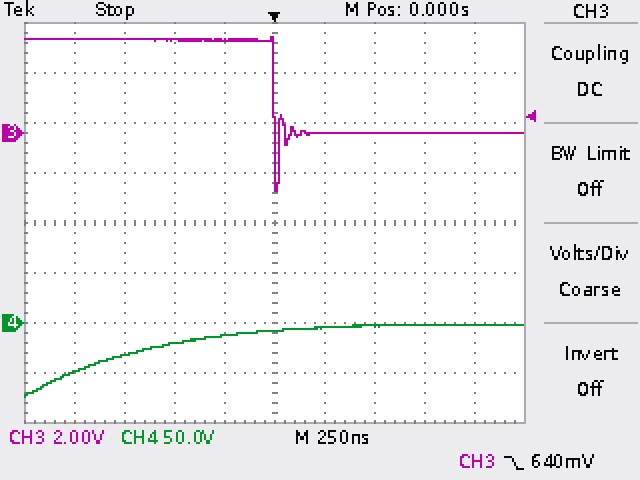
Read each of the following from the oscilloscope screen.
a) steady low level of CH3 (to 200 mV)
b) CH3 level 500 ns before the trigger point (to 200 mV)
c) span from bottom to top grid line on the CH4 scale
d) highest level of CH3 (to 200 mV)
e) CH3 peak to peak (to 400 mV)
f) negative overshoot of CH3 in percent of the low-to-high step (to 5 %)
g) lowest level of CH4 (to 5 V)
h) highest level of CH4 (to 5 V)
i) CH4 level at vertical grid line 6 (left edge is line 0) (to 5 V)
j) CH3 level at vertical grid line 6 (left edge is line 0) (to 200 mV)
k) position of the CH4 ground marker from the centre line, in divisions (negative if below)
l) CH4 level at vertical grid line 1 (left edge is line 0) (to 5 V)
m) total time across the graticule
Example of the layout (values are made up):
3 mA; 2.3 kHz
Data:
0.0 V; 3.8 V; 400 V; 3.8 V; 6.0 V; 60 %; -75 V; 0 V; -5 V; 0.0 V; -2.0 div; -50 V; 2.5 µs
